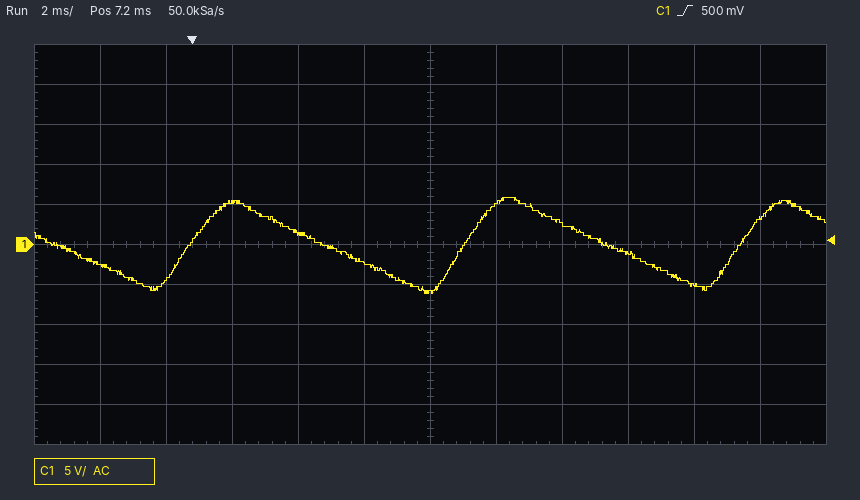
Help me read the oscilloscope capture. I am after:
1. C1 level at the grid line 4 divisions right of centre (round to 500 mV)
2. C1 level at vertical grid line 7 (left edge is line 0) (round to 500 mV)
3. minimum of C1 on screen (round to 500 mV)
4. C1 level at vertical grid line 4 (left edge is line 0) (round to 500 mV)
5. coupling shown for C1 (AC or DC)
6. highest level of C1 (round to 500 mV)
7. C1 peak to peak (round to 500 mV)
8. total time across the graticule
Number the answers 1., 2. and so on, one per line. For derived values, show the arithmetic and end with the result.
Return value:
1. -5.0 V
2. 5.0 V
3. -6.0 V
4. 1.5 V
5. AC
6. 6.0 V
7. 6.0 V − (-6.0 V) = 12.0 V
8. 24 ms
